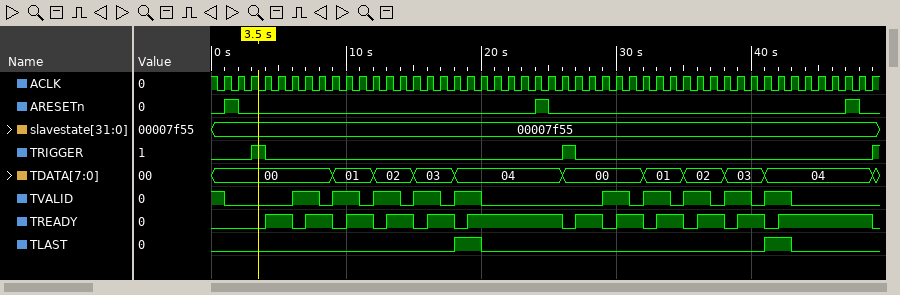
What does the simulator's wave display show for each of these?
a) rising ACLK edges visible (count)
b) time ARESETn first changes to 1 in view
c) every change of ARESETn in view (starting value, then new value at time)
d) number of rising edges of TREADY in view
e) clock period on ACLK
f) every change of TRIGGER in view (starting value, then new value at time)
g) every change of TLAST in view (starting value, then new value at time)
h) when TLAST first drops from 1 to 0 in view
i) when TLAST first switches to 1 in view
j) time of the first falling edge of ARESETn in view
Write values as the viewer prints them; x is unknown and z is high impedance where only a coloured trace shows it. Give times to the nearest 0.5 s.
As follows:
49
1 s
0, 1 at 1 s, 0 at 2 s, 1 at 24 s, 0 at 25 s, 1 at 47 s, 0 at 48 s
12
1 s
0, 1 at 3 s, 0 at 4 s, 1 at 26 s, 0 at 27 s, 1 at 49 s
0, 1 at 18 s, 0 at 20 s, 1 at 41 s, 0 at 43 s
20 s
18 s
2 s
